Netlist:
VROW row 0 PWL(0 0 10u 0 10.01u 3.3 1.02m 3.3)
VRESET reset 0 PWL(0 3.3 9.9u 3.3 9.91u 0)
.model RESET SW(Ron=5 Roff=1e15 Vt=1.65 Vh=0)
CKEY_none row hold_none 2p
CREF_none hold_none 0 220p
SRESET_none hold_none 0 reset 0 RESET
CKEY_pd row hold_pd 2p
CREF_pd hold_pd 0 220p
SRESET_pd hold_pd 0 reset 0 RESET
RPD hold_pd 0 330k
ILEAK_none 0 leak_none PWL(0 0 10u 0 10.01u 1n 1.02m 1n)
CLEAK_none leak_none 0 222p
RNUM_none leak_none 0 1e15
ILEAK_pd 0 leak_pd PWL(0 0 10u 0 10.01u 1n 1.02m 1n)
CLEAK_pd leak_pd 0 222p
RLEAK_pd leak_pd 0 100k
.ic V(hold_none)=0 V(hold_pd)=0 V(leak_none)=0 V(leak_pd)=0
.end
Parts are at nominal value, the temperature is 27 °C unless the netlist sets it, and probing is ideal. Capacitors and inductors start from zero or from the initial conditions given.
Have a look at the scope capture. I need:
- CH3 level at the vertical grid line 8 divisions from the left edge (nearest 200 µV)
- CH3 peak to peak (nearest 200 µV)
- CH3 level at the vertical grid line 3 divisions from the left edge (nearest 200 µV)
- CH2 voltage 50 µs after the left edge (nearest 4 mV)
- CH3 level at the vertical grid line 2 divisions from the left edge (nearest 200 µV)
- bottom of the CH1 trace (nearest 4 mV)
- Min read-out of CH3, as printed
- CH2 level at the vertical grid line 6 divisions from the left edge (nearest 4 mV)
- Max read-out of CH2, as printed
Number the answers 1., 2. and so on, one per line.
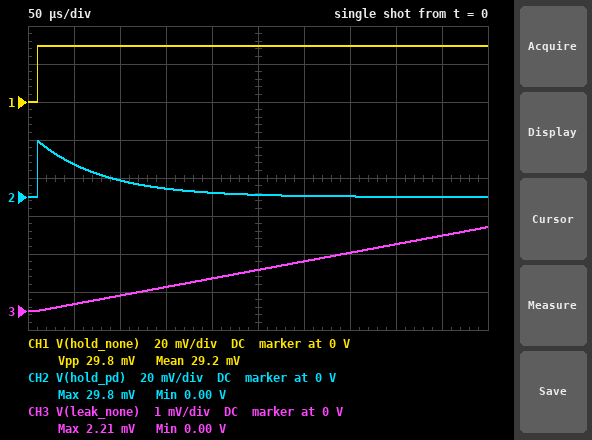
1. 1.8 mV
2. 2.2 mV
3. 600 µV
4. 16 mV
5. 400 µV
6. 0 V
7. 0.00 V
8. 0 V
9. 29.8 mV
